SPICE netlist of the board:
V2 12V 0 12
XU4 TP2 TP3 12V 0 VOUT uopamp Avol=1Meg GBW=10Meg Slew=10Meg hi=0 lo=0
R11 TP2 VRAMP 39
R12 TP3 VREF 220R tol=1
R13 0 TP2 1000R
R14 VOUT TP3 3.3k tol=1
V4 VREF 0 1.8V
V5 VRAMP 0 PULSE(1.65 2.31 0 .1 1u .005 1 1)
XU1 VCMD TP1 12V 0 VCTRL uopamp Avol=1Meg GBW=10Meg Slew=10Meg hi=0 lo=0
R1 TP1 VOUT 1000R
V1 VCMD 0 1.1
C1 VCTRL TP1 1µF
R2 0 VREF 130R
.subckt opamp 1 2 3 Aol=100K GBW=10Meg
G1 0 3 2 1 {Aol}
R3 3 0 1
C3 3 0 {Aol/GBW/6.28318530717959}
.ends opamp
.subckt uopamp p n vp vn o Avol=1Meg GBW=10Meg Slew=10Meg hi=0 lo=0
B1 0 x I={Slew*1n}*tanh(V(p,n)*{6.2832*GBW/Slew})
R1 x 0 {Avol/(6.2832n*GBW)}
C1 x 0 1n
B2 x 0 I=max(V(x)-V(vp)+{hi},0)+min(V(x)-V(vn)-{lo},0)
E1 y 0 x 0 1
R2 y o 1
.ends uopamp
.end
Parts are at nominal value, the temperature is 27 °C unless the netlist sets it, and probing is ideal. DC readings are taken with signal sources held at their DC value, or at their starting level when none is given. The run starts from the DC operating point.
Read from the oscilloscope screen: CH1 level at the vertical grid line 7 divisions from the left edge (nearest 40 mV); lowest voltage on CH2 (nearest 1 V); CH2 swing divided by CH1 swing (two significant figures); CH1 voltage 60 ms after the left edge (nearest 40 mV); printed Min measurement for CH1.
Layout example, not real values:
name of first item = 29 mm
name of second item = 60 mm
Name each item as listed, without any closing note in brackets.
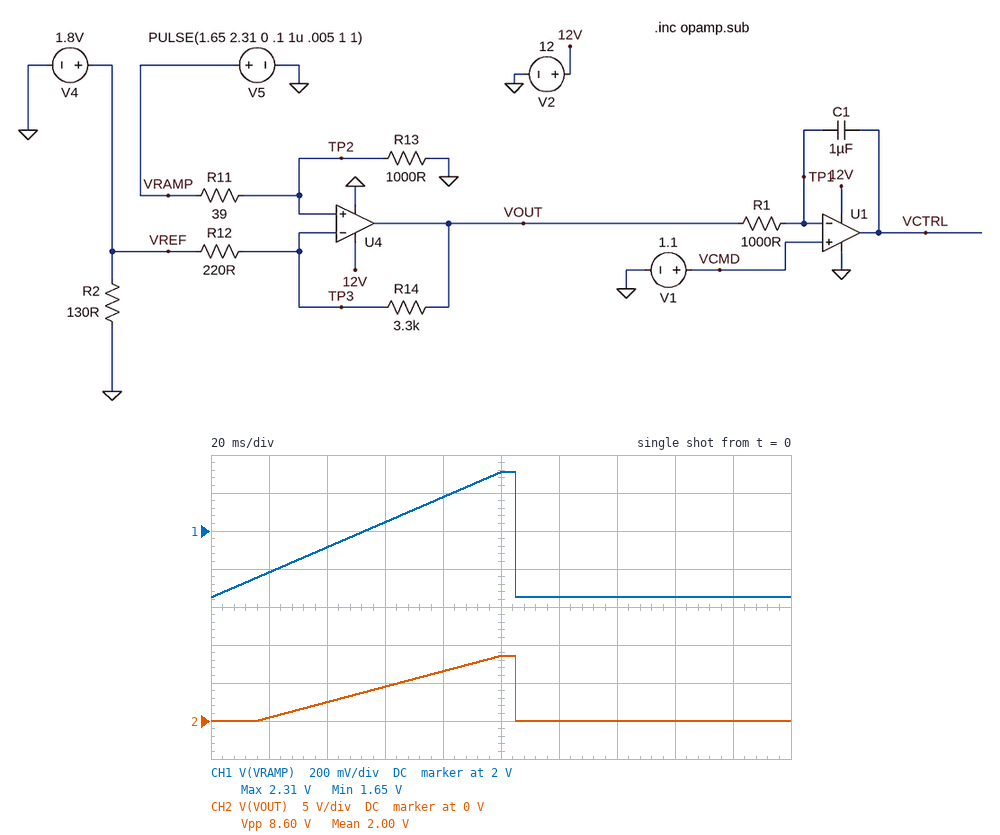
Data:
CH1 level at the vertical grid line 7 divisions from the left edge = 1.64 V
lowest voltage on CH2 = 0 V
CH2 swing divided by CH1 swing = 13
CH1 voltage 60 ms after the left edge = 2.04 V
printed Min measurement for CH1 = 1.65 V
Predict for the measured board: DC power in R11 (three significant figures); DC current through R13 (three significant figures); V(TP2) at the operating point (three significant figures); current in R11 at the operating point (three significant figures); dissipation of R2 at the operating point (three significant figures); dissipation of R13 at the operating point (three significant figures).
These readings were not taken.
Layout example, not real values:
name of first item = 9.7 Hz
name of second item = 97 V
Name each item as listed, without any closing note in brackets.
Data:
DC power in R11 = 98.4 µW
DC current through R13 = 1.59 mA
V(TP2) at the operating point = 1.59 V
current in R11 at the operating point = 1.59 mA
dissipation of R2 at the operating point = 24.9 mW
dissipation of R13 at the operating point = 2.52 mW
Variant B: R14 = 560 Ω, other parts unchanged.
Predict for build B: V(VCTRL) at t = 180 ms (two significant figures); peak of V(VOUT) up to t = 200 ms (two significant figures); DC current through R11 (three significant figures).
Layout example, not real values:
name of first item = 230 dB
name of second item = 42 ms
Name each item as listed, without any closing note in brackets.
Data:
V(VCTRL) at t = 180 ms = 3.7 V
peak of V(VOUT) up to t = 200 ms = 3.3 V
DC current through R11 = 1.59 mA
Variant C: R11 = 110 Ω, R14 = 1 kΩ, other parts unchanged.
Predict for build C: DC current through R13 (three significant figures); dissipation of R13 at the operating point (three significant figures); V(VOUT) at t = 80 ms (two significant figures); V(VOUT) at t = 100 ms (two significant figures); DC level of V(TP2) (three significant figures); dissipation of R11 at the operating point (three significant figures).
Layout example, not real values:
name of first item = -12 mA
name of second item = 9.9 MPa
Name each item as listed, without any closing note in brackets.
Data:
DC current through R13 = 1.49 mA
dissipation of R13 at the operating point = 2.21 mW
V(VOUT) at t = 80 ms = 2.7 V
V(VOUT) at t = 100 ms = 3.4 V
DC level of V(TP2) = 1.49 V
dissipation of R11 at the operating point = 243 µW
